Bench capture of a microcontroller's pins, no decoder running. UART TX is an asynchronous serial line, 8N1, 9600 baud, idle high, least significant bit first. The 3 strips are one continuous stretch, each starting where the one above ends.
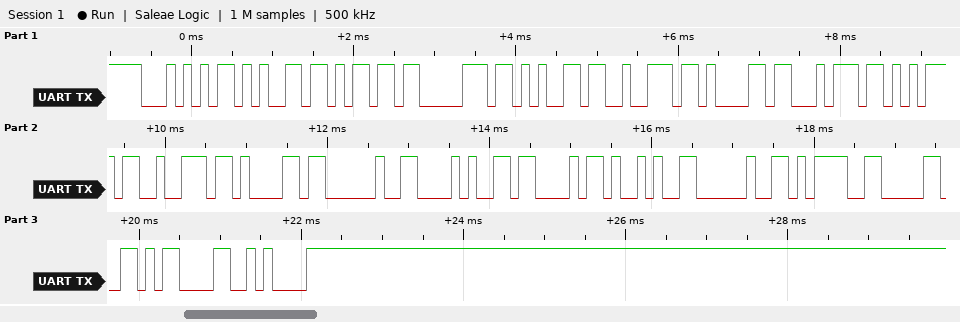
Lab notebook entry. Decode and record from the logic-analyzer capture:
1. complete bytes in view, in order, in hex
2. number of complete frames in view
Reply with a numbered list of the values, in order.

1. 0x54 0x65 0x6D 0x70 0x65 0x72 0x61 0x74 0x75 0x72 0x61 0x20 0x28 0x43 0x29 0x20 0x3D 0x30 0x0D 0x0A
2. 20
